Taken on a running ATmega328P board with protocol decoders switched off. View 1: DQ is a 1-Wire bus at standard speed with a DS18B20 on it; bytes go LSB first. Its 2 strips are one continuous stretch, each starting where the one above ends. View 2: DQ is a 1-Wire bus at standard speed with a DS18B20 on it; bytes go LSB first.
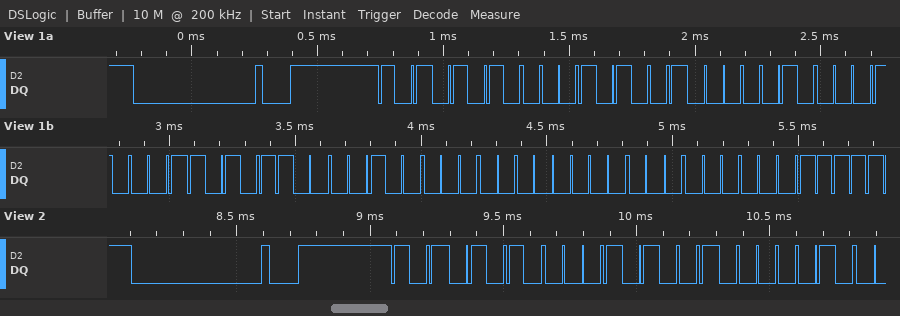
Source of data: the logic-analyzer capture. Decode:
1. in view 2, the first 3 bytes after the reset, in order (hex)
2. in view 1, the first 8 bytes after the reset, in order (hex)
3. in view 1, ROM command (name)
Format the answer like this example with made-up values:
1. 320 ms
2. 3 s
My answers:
1. 55 28 41
2. 55 28 41 88 35 04 00 00
3. Match ROM
